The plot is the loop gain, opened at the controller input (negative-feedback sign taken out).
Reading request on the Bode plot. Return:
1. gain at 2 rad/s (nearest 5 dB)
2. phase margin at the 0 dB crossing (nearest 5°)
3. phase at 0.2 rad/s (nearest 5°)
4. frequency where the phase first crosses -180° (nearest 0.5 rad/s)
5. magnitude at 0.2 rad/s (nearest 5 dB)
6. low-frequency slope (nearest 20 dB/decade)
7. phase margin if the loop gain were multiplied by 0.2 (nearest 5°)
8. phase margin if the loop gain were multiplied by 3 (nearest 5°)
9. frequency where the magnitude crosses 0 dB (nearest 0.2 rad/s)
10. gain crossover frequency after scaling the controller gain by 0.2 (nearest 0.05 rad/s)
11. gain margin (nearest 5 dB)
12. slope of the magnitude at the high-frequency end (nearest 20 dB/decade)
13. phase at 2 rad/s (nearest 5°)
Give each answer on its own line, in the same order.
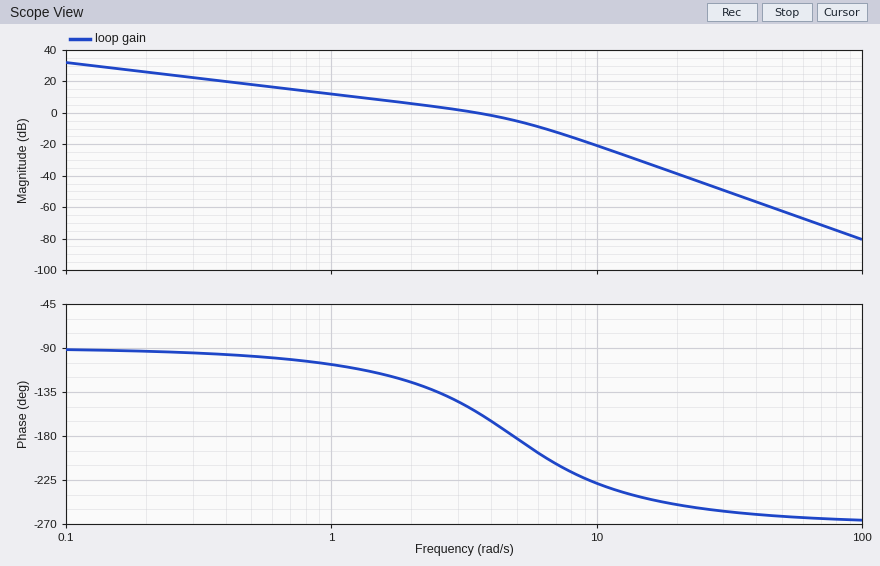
5 dB
25°
-95°
5.0 rad/s
25 dB
-20 dB/decade
75°
-20°
3.6 rad/s
0.80 rad/s
5 dB
-60 dB/decade
-125°
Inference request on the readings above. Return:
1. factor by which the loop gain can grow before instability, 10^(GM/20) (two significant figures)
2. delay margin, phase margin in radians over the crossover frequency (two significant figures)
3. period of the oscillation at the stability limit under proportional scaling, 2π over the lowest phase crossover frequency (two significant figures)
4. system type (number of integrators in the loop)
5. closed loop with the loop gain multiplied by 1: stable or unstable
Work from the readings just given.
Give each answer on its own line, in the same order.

1.8
0.12 s
1.3 s
1
stable
